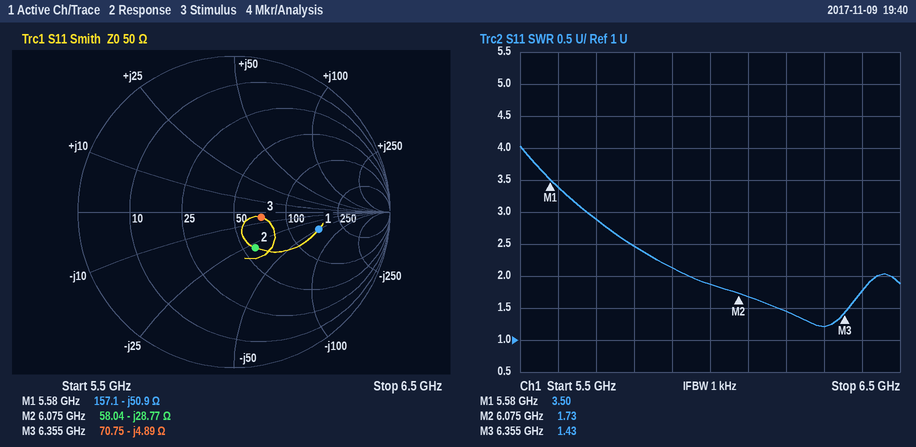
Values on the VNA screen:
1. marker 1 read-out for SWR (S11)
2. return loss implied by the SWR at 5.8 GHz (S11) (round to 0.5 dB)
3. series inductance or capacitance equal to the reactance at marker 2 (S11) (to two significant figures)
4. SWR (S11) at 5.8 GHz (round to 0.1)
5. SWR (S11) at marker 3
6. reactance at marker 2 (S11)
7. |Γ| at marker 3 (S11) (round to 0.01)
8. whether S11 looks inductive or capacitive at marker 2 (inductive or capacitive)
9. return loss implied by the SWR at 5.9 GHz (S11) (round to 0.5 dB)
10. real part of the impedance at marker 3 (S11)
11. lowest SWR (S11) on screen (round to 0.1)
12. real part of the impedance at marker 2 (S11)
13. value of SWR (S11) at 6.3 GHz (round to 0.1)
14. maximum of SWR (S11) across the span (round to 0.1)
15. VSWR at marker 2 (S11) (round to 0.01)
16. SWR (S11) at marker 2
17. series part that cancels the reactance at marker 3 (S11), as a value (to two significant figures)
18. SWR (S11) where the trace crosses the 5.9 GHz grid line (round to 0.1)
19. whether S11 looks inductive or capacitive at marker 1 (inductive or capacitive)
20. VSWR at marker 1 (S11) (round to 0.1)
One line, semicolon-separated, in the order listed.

3.50; 7.5 dB; 910 fF; 2.5; 1.43; -28.77 Ω; 0.18; capacitive; 9.0 dB; 70.75 Ω; 1.2; 58.04 Ω; 1.2; 4.0; 1.73; 1.73; 120 pH; 2.1; capacitive; 3.5
